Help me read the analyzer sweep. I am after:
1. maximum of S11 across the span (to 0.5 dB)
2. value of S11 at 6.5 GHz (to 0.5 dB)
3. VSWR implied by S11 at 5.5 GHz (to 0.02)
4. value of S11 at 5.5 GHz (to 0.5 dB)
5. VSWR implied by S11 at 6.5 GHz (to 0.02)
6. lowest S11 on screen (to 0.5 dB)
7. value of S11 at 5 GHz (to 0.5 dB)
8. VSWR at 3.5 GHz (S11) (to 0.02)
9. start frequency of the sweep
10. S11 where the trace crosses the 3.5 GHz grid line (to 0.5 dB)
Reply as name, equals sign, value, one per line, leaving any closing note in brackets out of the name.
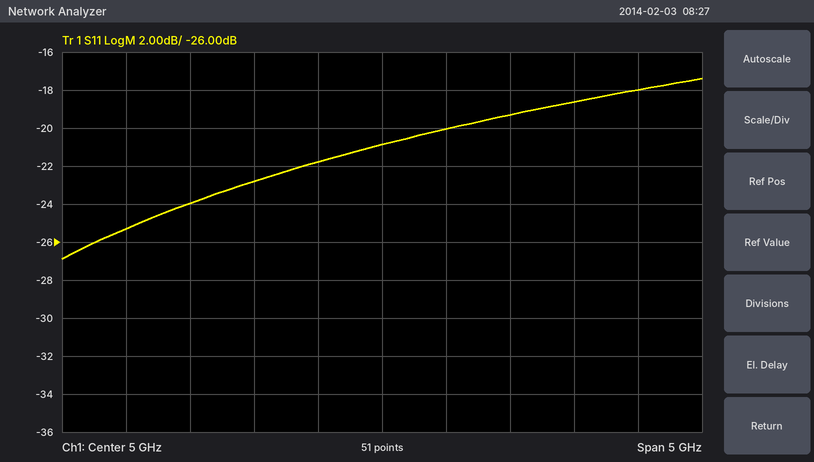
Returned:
maximum of S11 across the span = -17.5 dB
value of S11 at 6.5 GHz = -18.5 dB
VSWR implied by S11 at 5.5 GHz = 1.22
value of S11 at 5.5 GHz = -20.0 dB
VSWR implied by S11 at 6.5 GHz = 1.26
lowest S11 on screen = -27.0 dB
value of S11 at 5 GHz = -21.0 dB
VSWR at 3.5 GHz (S11) = 1.14
start frequency of the sweep = 2.5 GHz
S11 where the trace crosses the 3.5 GHz grid line = -24.0 dB
